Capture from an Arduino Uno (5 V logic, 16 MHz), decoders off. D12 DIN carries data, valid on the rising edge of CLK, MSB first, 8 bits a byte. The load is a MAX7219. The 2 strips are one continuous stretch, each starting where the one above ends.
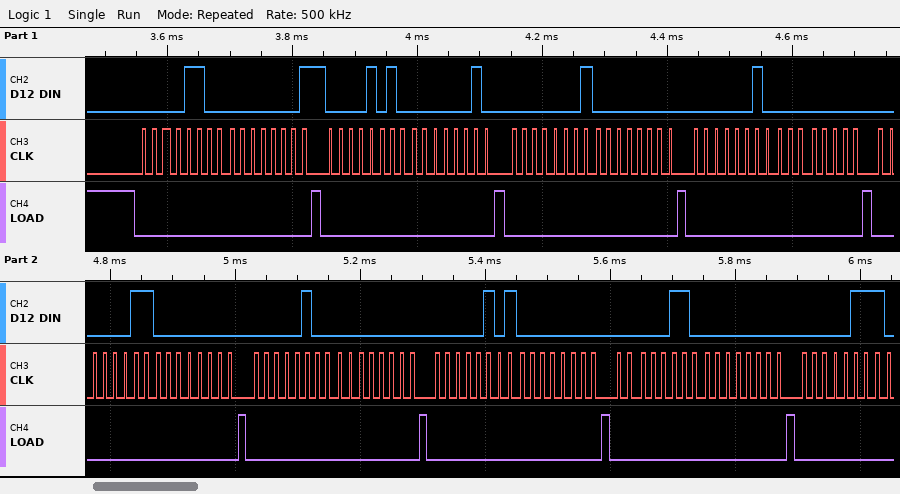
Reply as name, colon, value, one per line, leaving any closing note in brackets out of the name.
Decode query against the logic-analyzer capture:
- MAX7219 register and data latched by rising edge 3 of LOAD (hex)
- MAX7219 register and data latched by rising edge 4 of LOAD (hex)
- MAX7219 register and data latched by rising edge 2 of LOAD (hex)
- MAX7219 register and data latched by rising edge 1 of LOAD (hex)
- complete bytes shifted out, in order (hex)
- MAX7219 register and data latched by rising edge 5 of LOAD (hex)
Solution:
MAX7219 register and data latched by rising edge 3 of LOAD: register 0x1, data 0x00
MAX7219 register and data latched by rising edge 4 of LOAD: register 0x2, data 0x00
MAX7219 register and data latched by rising edge 2 of LOAD: register 0xA, data 0x02
MAX7219 register and data latched by rising edge 1 of LOAD: register 0xC, data 0x01
complete bytes shifted out, in order: 0C 01 0A 02 01 00 02 00 03 00 04 00 05 00 06 00 07
MAX7219 register and data latched by rising edge 5 of LOAD: register 0x3, data 0x00
